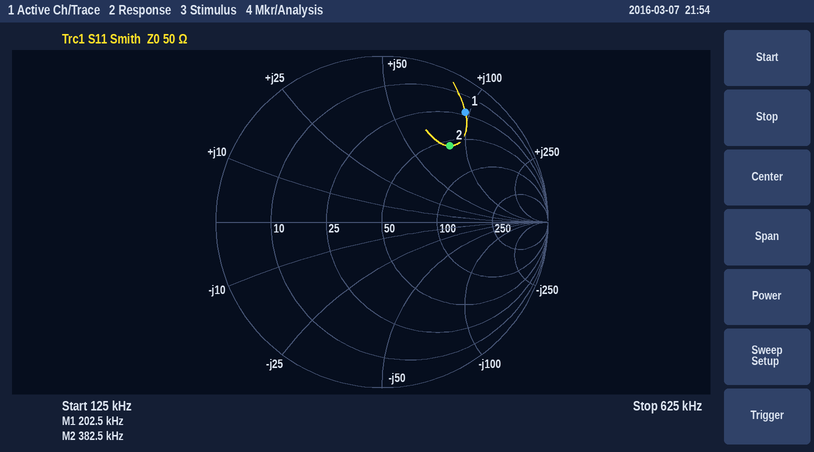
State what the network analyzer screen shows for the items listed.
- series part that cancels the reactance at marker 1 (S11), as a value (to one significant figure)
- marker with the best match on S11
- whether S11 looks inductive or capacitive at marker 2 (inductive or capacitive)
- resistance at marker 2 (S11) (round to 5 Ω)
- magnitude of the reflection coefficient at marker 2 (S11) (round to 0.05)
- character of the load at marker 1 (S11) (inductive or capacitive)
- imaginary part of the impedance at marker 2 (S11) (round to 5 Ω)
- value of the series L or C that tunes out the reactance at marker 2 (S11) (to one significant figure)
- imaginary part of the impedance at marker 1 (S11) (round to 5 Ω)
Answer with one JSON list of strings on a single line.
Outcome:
["8 nF", "marker 2", "inductive", "55 Ω", "0.60", "inductive", "+80 Ω", "5 nF", "+95 Ω"]
